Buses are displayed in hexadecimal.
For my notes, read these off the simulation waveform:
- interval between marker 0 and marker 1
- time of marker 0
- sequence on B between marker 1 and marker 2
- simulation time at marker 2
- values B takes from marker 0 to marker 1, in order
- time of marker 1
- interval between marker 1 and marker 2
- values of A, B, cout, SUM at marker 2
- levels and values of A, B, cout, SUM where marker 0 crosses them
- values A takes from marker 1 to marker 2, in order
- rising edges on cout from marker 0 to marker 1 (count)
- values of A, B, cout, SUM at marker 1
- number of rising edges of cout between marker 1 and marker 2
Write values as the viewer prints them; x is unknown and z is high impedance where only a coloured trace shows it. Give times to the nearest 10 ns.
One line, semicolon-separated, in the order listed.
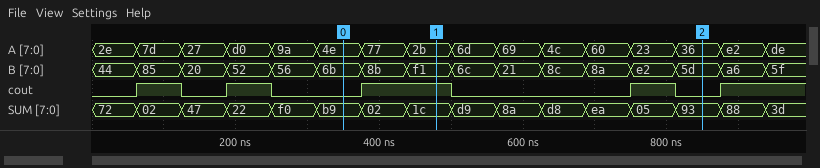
130 ns; 350 ns; f1, 6c, 21, 8c, 8a, e2, 5d; 850 ns; 6b, 8b, f1; 480 ns; 370 ns; A=36, B=5d, cout=0, SUM=93; A=4e, B=6b, cout=0, SUM=b9; 2b, 6d, 69, 4c, 60, 23, 36; 1; A=2b, B=f1, cout=1, SUM=1c; 1
